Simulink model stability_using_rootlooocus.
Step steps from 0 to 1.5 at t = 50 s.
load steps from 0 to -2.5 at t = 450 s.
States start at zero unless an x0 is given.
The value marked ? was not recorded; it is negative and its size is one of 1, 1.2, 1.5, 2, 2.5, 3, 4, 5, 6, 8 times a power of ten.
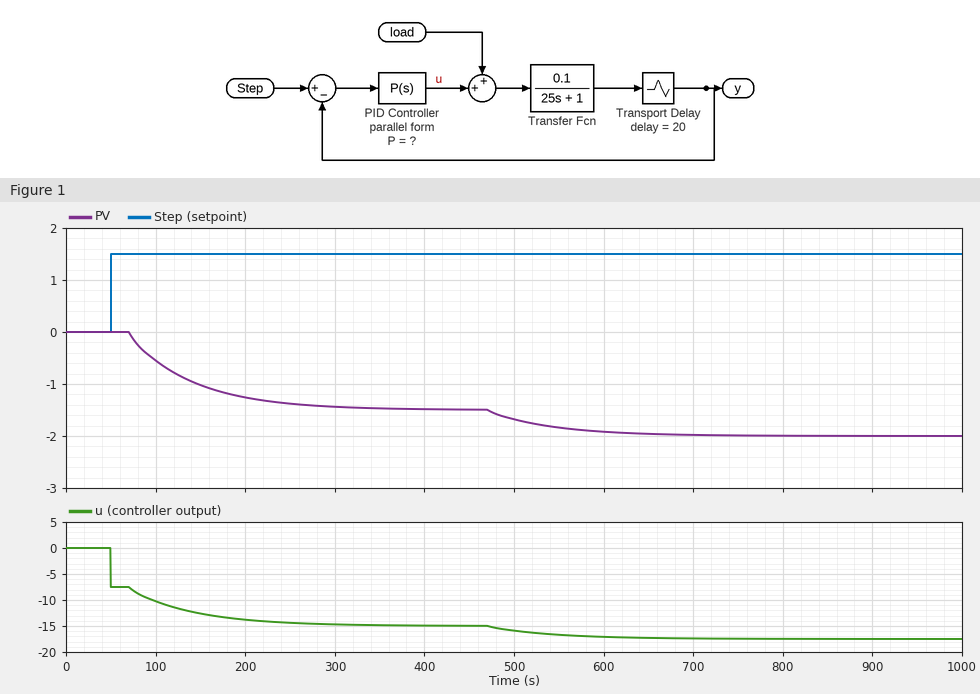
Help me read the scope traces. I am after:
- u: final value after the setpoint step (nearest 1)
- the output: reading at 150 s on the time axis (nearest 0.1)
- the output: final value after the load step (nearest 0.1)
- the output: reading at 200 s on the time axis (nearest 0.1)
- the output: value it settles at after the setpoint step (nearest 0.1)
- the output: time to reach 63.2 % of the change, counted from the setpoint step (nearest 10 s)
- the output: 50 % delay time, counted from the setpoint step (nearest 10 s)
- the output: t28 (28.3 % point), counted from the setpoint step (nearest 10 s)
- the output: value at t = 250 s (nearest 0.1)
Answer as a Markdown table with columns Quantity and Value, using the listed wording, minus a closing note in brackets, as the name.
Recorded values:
| Quantity | Value |
|---|---|
| u: final value after the setpoint step | -15 |
| the output: reading at 150 s on the time axis | -1.0 |
| the output: final value after the load step | -2.0 |
| the output: reading at 200 s on the time axis | -1.3 |
| the output: value it settles at after the setpoint step | -1.5 |
| the output: time to reach 63.2 % of the change, counted from the setpoint step | 90 s |
| the output: 50 % delay time, counted from the setpoint step | 70 s |
| the output: t28 (28.3 % point), counted from the setpoint step | 40 s |
| the output: value at t = 250 s | -1.4 |
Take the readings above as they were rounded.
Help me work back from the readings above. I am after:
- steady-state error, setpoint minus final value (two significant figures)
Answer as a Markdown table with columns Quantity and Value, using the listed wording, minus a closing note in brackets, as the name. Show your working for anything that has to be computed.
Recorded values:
| Quantity | Value |
|---|---|
| steady-state error, setpoint minus final value | 1.5 - (-1.5) = 3.0 |
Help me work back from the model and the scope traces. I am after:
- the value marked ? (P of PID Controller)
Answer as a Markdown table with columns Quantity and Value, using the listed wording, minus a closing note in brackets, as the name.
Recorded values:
| Quantity | Value |
|---|---|
| the value marked ? | -5 |
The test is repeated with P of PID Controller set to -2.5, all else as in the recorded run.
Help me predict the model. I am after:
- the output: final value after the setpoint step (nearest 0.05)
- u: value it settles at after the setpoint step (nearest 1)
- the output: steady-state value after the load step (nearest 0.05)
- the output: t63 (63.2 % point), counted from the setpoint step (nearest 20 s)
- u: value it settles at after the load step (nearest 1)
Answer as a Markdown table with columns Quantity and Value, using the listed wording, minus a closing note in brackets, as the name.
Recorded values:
| Quantity | Value |
|---|---|
| the output: final value after the setpoint step | -0.50 |
| u: value it settles at after the setpoint step | -5 |
| the output: steady-state value after the load step | -0.85 |
| the output: t63 (63.2 % point), counted from the setpoint step | 60 s |
| u: value it settles at after the load step | -6 |
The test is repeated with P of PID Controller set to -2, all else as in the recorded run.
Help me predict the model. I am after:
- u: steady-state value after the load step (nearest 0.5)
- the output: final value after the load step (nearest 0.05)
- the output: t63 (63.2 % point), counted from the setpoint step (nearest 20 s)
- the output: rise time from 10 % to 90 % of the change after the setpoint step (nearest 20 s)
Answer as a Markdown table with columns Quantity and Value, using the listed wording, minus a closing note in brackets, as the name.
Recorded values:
| Quantity | Value |
|---|---|
| u: steady-state value after the load step | -4.5 |
| the output: final value after the load step | -0.70 |
| the output: t63 (63.2 % point), counted from the setpoint step | 60 s |
| the output: rise time from 10 % to 90 % of the change after the setpoint step | 80 s |
